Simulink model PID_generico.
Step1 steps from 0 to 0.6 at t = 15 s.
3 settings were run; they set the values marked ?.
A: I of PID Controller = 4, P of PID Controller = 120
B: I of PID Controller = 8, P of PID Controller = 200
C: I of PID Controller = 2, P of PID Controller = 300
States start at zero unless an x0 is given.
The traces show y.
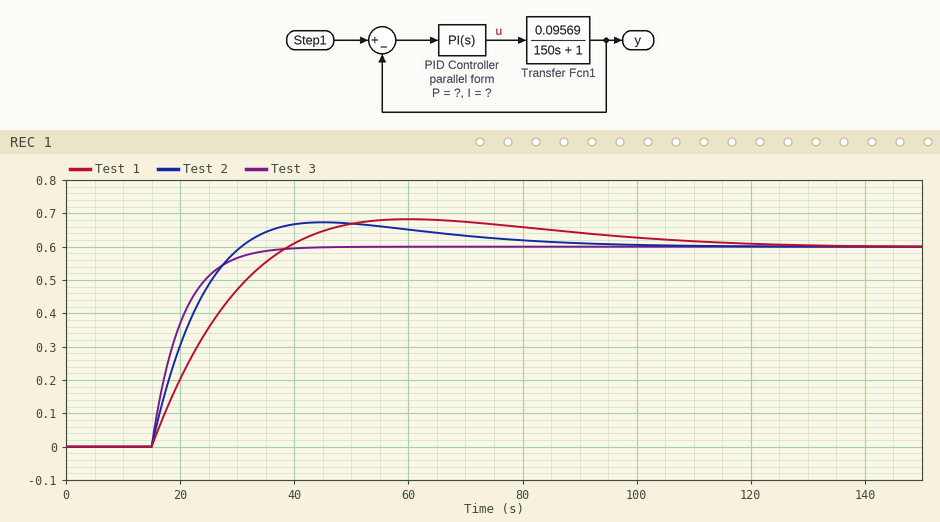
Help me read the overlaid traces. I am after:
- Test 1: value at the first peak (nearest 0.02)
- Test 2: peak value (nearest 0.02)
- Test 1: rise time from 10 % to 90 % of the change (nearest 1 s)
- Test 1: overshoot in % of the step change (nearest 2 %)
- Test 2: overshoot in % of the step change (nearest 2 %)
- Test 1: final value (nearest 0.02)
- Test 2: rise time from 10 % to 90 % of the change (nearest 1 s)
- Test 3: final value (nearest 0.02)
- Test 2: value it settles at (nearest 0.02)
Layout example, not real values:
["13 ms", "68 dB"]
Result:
["0.68", "0.68", "18 s", "14 %", "12 %", "0.60", "11 s", "0.60", "0.60"]
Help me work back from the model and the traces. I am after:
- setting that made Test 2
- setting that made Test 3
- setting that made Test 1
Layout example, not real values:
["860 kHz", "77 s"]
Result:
["B", "C", "A"]
